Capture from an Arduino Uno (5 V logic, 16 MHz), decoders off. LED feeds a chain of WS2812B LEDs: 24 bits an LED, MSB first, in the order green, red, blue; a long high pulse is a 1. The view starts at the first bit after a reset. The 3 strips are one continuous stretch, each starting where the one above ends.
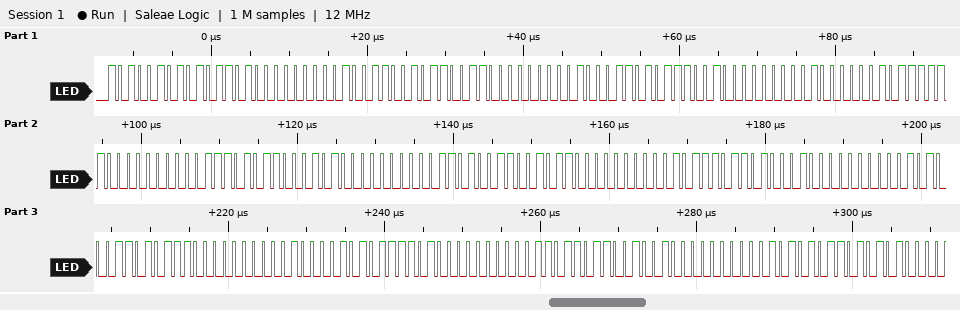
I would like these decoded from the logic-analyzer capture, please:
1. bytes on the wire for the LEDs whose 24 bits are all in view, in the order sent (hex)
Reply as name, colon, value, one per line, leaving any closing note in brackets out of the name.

bytes on the wire for the LEDs whose 24 bits are all in view, in the order sent: A5 5A 00 99 66 00 8D 72 00 81 7E 00 75 8A 00 69 96 00 5D A2 00 51 AE 00 42 BD 00 36 C9 00
